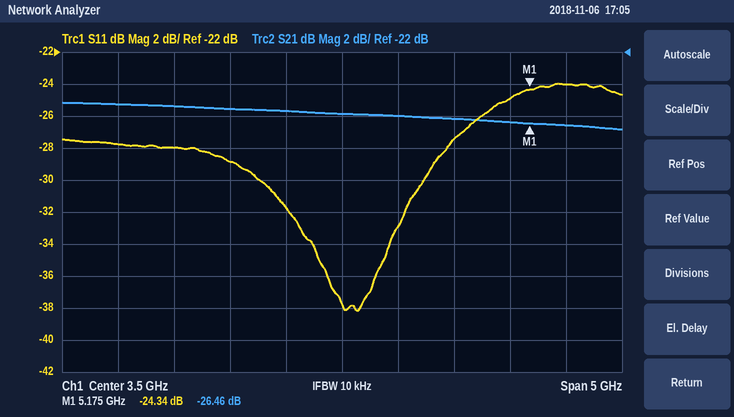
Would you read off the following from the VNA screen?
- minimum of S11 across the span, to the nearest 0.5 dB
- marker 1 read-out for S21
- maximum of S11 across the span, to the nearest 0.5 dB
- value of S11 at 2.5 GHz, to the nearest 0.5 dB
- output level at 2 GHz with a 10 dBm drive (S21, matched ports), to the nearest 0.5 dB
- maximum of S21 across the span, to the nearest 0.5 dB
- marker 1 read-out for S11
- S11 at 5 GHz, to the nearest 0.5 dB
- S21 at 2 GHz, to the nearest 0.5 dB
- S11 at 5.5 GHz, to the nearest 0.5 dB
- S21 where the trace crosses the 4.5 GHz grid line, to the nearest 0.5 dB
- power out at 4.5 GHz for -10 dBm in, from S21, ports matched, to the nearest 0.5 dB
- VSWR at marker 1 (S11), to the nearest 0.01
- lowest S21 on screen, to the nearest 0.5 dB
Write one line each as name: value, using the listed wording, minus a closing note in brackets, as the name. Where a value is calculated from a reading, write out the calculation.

minimum of S11 across the span, to the nearest 0.5 dB: -38.0 dB
marker 1 read-out for S21: -26.46 dB
maximum of S11 across the span, to the nearest 0.5 dB: -24.0 dB
value of S11 at 2.5 GHz, to the nearest 0.5 dB: -29.0 dB
output level at 2 GHz with a 10 dBm drive (S21, matched ports), to the nearest 0.5 dB: 10 dBm + (-25.5 dB) = -15.5 dBm
maximum of S21 across the span, to the nearest 0.5 dB: -25.0 dB
marker 1 read-out for S11: -24.34 dB
S11 at 5 GHz, to the nearest 0.5 dB: -25.0 dB
S21 at 2 GHz, to the nearest 0.5 dB: -25.5 dB
S11 at 5.5 GHz, to the nearest 0.5 dB: -24.0 dB
S21 where the trace crosses the 4.5 GHz grid line, to the nearest 0.5 dB: -26.0 dB
power out at 4.5 GHz for -10 dBm in, from S21, ports matched, to the nearest 0.5 dB: -10 dBm + (-26.0 dB) = -36.0 dBm
VSWR at marker 1 (S11), to the nearest 0.01: (1 + 0.0607)/(1 − 0.0607) ≈ 1.13
lowest S21 on screen, to the nearest 0.5 dB: -27.0 dB
